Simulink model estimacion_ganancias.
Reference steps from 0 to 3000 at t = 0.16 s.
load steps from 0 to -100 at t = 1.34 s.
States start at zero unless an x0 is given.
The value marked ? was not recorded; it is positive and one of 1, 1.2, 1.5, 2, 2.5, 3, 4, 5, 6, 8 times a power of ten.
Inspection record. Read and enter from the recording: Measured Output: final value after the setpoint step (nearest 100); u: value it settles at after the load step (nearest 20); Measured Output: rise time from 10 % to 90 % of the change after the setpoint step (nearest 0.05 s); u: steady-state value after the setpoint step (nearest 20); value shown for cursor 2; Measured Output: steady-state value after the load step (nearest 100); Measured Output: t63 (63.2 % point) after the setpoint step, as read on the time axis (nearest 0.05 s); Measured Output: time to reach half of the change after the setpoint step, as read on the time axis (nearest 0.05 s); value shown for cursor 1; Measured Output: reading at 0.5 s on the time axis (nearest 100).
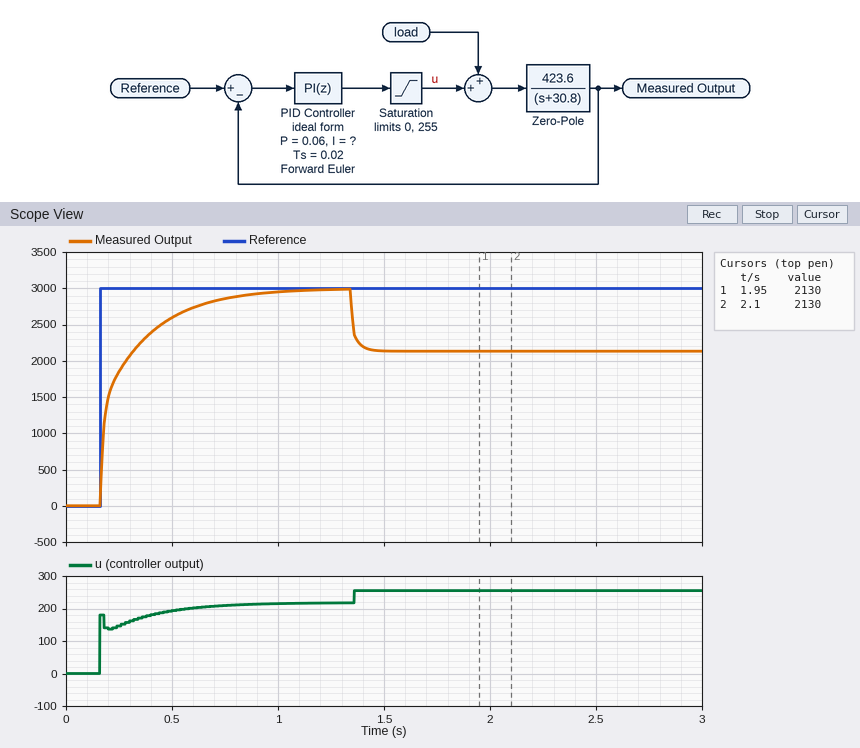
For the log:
3000
260
0.40 s
220
2130
2100
0.25 s
0.20 s
2130
2600
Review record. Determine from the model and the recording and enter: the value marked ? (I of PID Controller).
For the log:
8
